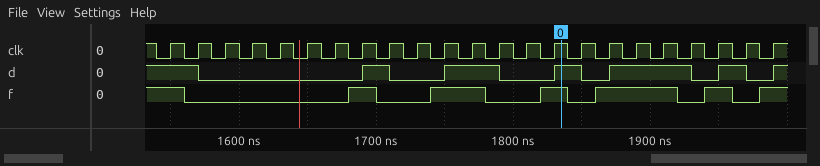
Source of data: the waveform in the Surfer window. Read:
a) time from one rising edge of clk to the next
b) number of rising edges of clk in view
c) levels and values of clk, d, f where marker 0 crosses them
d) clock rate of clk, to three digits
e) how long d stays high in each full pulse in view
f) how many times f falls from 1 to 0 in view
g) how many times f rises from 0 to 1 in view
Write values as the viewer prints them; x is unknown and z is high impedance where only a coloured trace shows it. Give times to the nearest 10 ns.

20 ns
23
clk=1, d=1, f=1
50.0 MHz
20 ns, 40 ns, 20 ns, 60 ns, 20 ns
6
6
